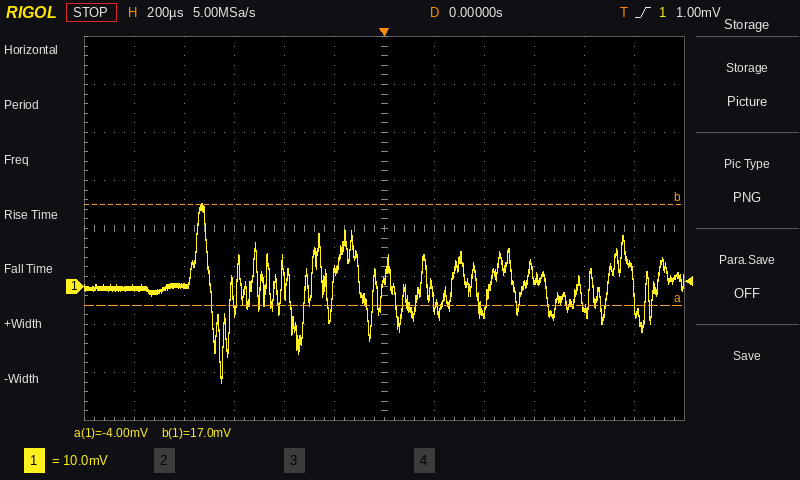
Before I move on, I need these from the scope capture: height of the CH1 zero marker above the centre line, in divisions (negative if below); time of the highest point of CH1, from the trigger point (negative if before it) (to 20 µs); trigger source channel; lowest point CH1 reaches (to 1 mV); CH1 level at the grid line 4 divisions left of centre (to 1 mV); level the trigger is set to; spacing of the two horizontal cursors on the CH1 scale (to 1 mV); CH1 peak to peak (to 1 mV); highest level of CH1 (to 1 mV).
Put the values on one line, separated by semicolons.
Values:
-1.2 div; -720 µs; CH1; -20 mV; 0 mV; 1.00 mV; 21 mV; 37 mV; 17 mV
